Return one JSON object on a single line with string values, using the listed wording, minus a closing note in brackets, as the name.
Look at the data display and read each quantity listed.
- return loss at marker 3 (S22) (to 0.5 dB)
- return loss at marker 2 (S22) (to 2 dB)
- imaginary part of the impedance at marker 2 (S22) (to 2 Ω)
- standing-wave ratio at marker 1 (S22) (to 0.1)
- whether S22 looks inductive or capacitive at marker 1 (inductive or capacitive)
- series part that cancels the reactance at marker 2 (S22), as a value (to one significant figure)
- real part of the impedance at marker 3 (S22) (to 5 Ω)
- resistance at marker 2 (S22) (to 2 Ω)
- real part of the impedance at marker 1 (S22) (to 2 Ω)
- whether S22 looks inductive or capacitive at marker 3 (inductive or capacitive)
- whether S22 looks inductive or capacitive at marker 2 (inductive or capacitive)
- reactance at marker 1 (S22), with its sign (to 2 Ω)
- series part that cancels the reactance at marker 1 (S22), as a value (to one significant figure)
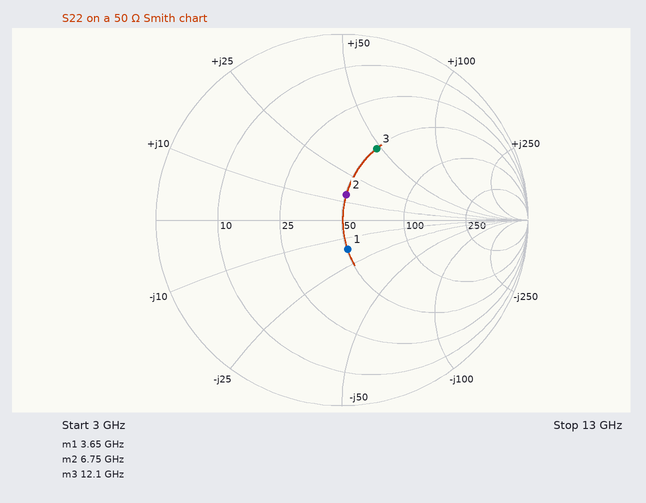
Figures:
{"return loss at marker 3 (S22)": "7.5 dB", "return loss at marker 2 (S22)": "18 dB", "imaginary part of the impedance at marker 2 (S22)": "+14 Ω", "standing-wave ratio at marker 1 (S22)": "1.4", "whether S22 looks inductive or capacitive at marker 1": "capacitive", "series part that cancels the reactance at marker 2 (S22), as a value": "2 pF", "real part of the impedance at marker 3 (S22)": "50 Ω", "resistance at marker 2 (S22)": "50 Ω", "real part of the impedance at marker 1 (S22)": "50 Ω", "whether S22 looks inductive or capacitive at marker 3": "inductive", "whether S22 looks inductive or capacitive at marker 2": "inductive", "reactance at marker 1 (S22), with its sign": "-16 Ω", "series part that cancels the reactance at marker 1 (S22), as a value": "700 pH"}
